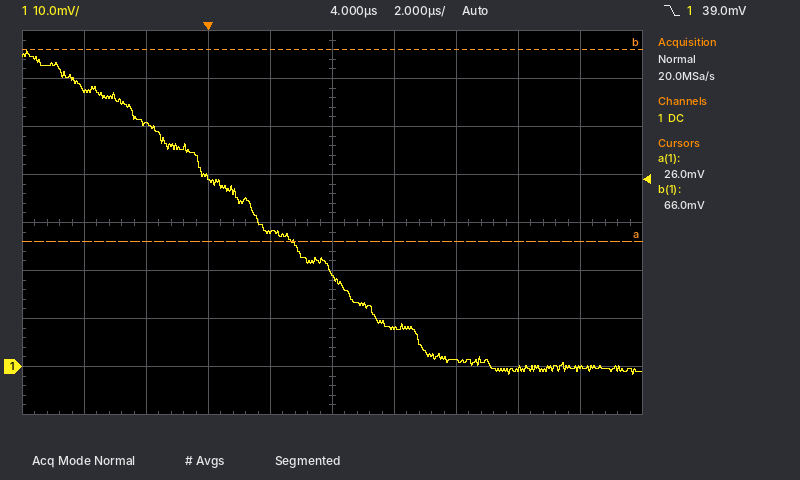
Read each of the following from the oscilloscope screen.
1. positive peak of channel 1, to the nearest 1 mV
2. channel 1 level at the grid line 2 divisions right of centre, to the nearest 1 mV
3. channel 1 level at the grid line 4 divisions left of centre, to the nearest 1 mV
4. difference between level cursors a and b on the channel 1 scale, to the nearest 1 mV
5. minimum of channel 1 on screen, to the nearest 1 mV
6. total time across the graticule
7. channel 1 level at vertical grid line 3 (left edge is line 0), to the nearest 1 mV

66 mV
1 mV
58 mV
40 mV
-2 mV
20 µs
39 mV
